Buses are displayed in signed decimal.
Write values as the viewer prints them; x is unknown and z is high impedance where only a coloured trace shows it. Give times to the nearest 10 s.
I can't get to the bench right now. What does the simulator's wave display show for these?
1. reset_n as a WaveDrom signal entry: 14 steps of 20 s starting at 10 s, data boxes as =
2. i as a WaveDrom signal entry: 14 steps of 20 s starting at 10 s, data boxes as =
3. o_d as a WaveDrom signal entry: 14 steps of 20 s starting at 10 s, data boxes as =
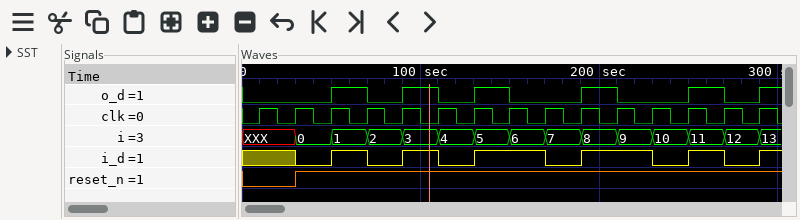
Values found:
{name: 'reset_n', wave: '01............'}
{name: 'i', wave: 'x=============', data: '0 1 2 3 4 5 6 7 8 9 10 11 12'}
{name: 'o_d', wave: '0.101010.10.10'}
